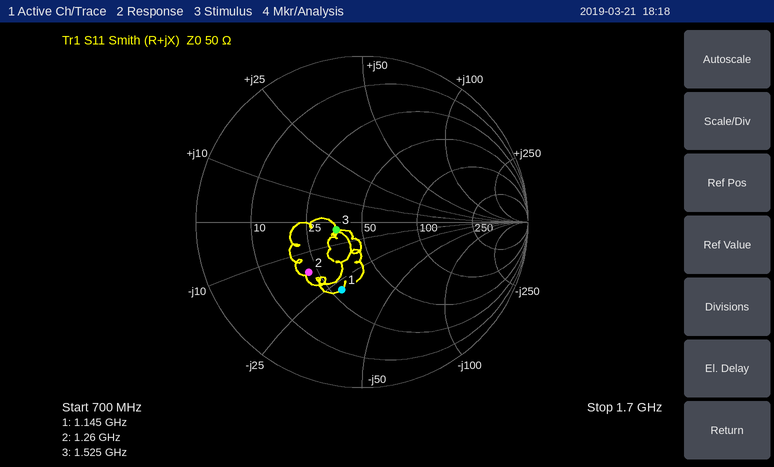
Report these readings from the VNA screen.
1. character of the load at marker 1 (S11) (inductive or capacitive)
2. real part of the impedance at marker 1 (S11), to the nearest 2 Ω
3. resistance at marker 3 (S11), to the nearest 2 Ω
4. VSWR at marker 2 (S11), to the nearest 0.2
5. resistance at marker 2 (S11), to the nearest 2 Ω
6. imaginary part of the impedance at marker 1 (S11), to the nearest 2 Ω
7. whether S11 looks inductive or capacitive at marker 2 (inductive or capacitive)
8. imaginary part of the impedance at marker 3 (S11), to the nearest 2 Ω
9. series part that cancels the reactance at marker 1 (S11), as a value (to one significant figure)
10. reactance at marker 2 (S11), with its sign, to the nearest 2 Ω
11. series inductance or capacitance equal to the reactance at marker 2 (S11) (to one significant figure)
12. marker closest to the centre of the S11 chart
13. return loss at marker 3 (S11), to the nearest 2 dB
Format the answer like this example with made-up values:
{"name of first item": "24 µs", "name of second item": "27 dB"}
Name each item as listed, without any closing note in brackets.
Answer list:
{"character of the load at marker 1 (S11)": "capacitive", "real part of the impedance at marker 1 (S11), to the nearest 2 Ω": "28 Ω", "resistance at marker 3 (S11), to the nearest 2 Ω": "36 Ω", "VSWR at marker 2 (S11), to the nearest 0.2": "2.6", "resistance at marker 2 (S11), to the nearest 2 Ω": "22 Ω", "imaginary part of the impedance at marker 1 (S11), to the nearest 2 Ω": "-28 Ω", "whether S11 looks inductive or capacitive at marker 2": "capacitive", "imaginary part of the impedance at marker 3 (S11), to the nearest 2 Ω": "-4 Ω", "series part that cancels the reactance at marker 1 (S11), as a value": "4 nH", "reactance at marker 2 (S11), with its sign, to the nearest 2 Ω": "-16 Ω", "series inductance or capacitance equal to the reactance at marker 2 (S11)": "8 pF", "marker closest to the centre of the S11 chart": "marker 3", "return loss at marker 3 (S11), to the nearest 2 dB": "16 dB"}
